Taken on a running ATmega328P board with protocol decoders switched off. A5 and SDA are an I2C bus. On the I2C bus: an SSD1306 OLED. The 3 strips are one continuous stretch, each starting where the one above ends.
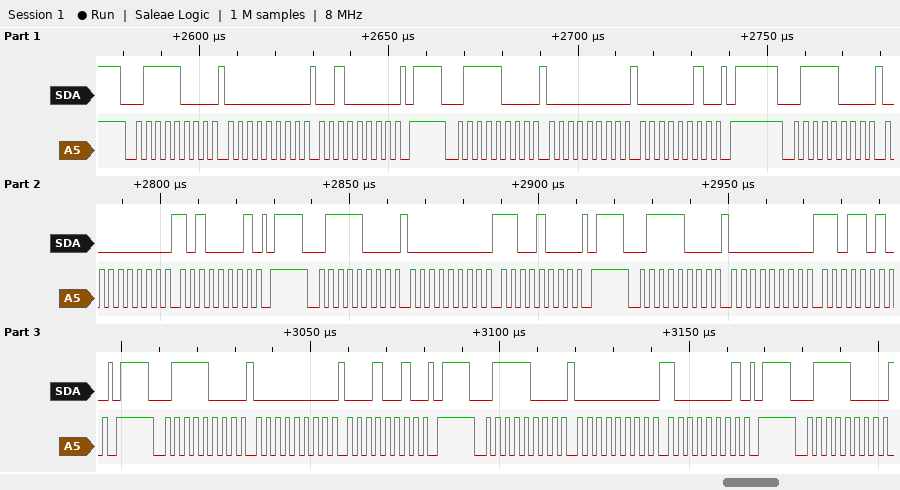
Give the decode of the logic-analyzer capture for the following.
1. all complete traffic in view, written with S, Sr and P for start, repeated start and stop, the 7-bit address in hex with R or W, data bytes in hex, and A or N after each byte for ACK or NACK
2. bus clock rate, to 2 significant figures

S 3CW A 00 A 20 A P S 3CW A 00 A 02 A P S 3CW A 00 A A1 A P S 3CW A 00 A C8 A P S 3CW A 00 A DA A P S 3CW A 00 A 12 A P S 3CW A 00 A 81 A P S 3CW A
400 kHz
